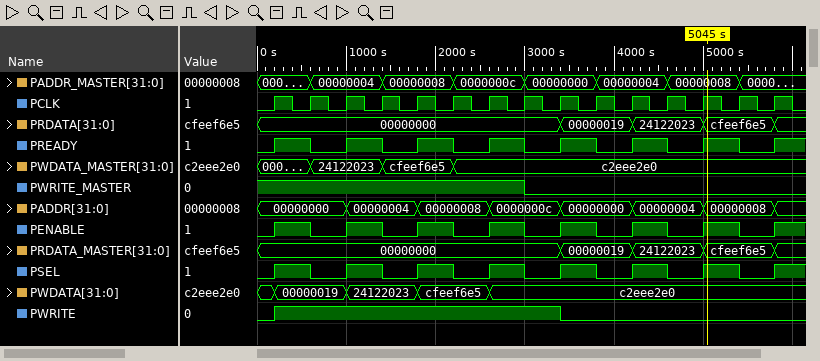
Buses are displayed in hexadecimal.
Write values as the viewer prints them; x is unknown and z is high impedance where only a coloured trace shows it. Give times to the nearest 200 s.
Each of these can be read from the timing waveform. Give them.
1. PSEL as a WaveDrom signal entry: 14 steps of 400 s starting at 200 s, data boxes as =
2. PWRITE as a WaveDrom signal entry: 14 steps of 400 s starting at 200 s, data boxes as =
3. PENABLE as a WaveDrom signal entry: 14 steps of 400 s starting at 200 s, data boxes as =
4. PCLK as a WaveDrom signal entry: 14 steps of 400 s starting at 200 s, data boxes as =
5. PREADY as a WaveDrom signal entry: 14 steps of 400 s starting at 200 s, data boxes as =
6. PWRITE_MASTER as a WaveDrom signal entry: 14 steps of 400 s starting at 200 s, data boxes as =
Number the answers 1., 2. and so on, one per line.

1. {name: 'PSEL', wave: '10101010101010'}
2. {name: 'PWRITE', wave: '1.......0.....'}
3. {name: 'PENABLE', wave: '10101010101010'}
4. {name: 'PCLK', wave: 'p.............'}
5. {name: 'PREADY', wave: '10101010101010'}
6. {name: 'PWRITE_MASTER', wave: '1......0......'}
